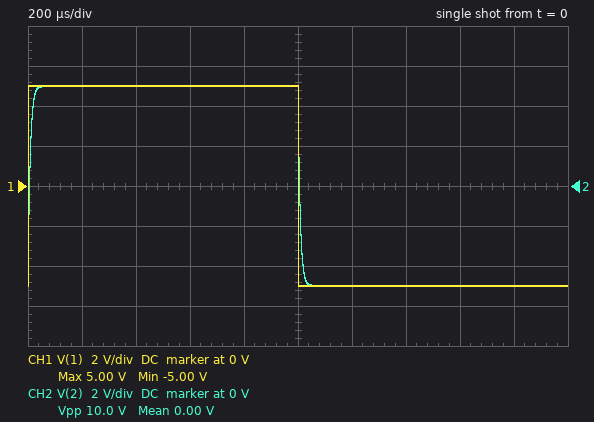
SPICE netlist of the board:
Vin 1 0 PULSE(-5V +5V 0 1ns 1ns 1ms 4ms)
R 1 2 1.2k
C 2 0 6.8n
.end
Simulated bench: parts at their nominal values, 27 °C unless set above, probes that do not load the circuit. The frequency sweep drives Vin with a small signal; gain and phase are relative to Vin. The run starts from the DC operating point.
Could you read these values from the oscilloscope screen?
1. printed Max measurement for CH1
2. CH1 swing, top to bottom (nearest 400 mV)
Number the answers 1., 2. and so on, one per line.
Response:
1. 5.00 V
2. 10.0 V
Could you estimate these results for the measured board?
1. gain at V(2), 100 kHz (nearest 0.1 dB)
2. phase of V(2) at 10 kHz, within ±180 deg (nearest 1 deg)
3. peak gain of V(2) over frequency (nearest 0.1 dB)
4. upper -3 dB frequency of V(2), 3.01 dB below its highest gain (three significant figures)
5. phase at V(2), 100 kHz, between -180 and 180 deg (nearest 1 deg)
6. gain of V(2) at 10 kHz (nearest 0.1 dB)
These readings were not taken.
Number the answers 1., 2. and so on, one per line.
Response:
1. -14.4 dB
2. -27 deg
3. 0 dB
4. 19.5 kHz
5. -79 deg
6. -1.0 dB
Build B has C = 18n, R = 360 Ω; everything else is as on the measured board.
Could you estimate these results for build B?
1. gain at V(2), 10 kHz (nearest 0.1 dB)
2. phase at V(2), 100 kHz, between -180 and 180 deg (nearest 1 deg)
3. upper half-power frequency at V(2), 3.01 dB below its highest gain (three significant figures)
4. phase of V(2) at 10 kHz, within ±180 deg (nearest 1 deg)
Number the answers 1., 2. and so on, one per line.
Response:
1. -0.7 dB
2. -76 deg
3. 24.6 kHz
4. -22 deg
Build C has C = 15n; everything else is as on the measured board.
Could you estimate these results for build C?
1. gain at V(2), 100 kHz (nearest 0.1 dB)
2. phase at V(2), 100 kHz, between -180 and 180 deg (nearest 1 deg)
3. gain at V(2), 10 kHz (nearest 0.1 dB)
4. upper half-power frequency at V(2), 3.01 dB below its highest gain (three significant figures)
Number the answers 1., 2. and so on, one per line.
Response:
1. -21.1 dB
2. -85 deg
3. -3.6 dB
4. 8.84 kHz
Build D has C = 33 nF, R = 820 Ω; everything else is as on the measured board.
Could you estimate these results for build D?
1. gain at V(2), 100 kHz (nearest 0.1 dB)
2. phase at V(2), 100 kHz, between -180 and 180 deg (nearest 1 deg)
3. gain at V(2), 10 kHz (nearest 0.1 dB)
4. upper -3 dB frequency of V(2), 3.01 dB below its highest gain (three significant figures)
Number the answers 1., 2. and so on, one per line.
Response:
1. -24.6 dB
2. -87 deg
3. -5.9 dB
4. 5.88 kHz
